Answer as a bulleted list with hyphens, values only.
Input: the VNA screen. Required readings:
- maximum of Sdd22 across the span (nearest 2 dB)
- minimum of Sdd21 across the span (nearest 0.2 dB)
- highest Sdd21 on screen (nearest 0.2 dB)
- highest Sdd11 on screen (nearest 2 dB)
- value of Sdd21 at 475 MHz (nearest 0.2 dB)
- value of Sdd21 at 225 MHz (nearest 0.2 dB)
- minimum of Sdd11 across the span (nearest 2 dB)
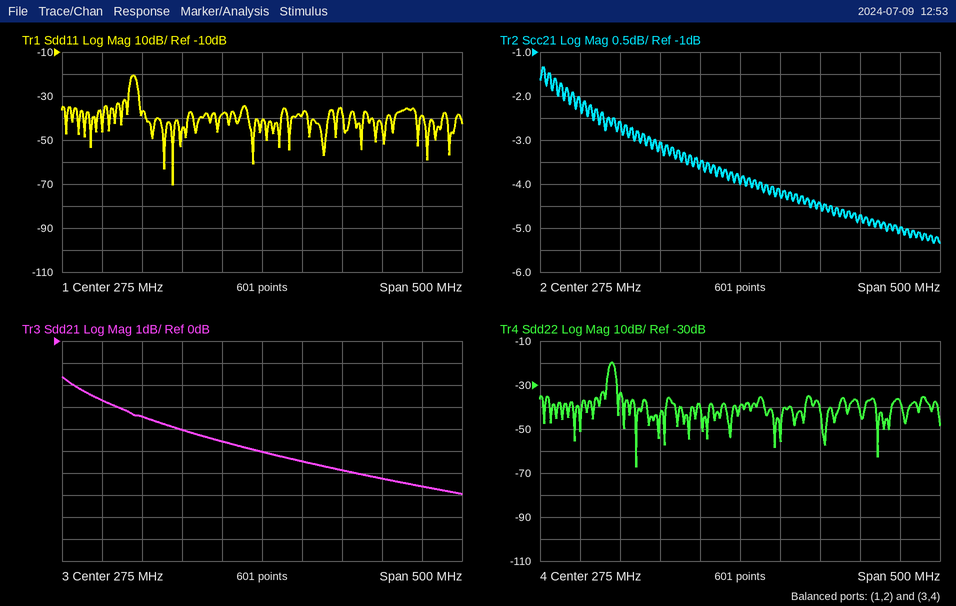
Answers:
- -20 dB
- -7.0 dB
- -1.6 dB
- -20 dB
- -6.6 dB
- -4.6 dB
- -70 dB
